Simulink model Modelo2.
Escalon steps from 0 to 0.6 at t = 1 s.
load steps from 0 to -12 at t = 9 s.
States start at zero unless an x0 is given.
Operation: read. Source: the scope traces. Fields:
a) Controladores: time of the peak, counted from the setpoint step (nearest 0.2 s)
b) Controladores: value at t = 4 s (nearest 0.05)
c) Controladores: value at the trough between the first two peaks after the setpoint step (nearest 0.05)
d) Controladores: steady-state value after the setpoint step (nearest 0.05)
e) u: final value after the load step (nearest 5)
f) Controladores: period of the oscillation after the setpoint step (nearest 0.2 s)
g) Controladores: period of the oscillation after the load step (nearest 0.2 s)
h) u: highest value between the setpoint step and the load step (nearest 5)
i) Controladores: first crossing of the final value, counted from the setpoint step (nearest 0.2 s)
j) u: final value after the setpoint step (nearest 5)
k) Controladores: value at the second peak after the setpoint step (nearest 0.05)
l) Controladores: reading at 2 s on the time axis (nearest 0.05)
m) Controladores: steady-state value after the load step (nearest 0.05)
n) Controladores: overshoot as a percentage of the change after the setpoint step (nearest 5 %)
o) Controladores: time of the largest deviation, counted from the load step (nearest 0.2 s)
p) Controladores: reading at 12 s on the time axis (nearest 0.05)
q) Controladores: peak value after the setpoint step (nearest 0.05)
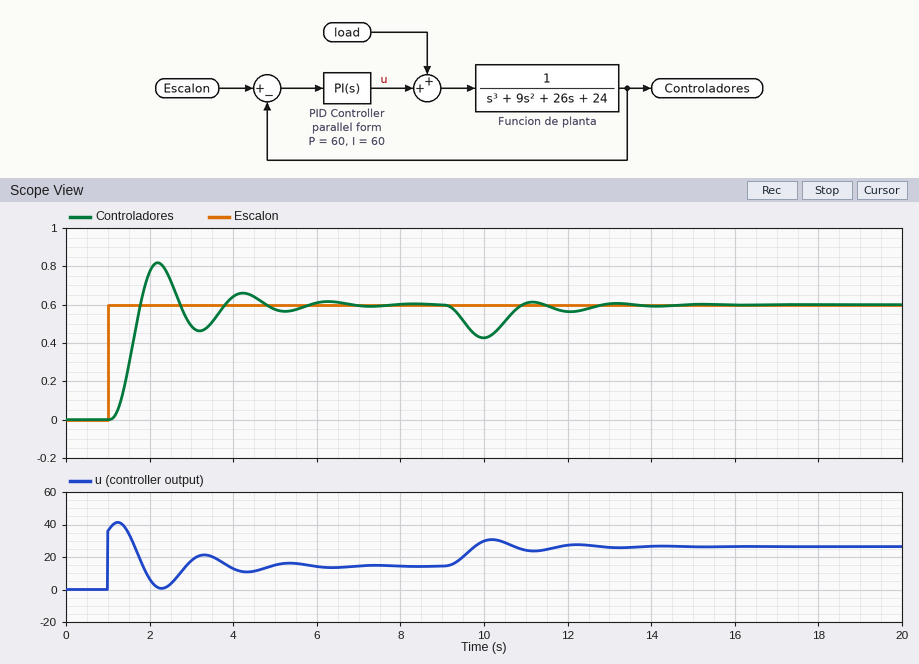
1.2 s
0.65
0.45
0.60
25
2.0 s
2.0 s
40
0.8 s
15
0.65
0.75
0.60
35 %
1.0 s
0.55
0.80
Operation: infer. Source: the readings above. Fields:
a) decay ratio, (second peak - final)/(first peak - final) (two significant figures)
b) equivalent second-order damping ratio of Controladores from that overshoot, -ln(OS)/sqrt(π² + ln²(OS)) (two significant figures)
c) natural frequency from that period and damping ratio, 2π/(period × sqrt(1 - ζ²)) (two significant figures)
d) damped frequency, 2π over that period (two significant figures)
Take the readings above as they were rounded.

0.25
0.32
3.3 rad/s
3.1 rad/s
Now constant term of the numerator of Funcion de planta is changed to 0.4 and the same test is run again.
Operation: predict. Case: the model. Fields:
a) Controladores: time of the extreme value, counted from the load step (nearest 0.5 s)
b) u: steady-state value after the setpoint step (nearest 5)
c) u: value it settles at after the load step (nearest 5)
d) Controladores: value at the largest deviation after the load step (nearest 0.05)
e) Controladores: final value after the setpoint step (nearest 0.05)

1.5 s
35
50
0.50
0.60
